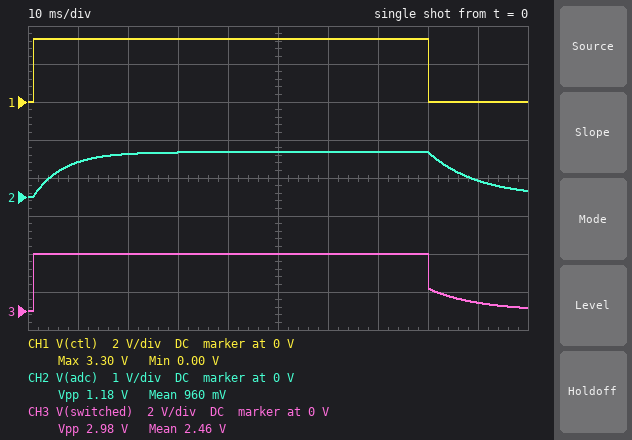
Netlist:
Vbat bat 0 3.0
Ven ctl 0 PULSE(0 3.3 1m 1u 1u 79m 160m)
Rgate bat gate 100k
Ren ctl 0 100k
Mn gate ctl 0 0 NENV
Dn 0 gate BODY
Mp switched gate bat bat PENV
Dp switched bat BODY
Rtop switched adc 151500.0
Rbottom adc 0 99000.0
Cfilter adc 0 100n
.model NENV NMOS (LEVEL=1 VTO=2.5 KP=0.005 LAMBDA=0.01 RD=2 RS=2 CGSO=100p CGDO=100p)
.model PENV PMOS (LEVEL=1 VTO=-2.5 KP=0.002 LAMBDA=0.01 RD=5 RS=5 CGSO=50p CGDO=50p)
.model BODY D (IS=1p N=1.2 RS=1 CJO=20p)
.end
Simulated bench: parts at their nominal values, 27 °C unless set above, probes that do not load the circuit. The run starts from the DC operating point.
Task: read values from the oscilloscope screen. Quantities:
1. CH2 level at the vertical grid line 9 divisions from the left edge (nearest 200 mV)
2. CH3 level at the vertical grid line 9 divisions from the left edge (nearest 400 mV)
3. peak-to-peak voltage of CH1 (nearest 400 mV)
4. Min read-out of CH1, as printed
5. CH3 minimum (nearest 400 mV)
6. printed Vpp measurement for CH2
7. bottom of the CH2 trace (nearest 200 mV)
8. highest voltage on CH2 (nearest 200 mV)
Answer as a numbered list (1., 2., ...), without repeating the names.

1. 400 mV
2. 400 mV
3. 3.2 V
4. 0.00 V
5. 0 V
6. 1.18 V
7. 0 V
8. 1.2 V
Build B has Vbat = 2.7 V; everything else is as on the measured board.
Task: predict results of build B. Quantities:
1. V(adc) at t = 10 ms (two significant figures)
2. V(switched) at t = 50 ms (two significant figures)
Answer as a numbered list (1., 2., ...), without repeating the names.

1. 820 mV
2. 2.7 V
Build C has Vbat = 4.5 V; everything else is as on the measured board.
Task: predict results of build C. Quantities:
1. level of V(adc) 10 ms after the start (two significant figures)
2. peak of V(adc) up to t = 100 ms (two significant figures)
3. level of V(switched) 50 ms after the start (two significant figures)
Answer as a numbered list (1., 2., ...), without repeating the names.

1. 1.4 V
2. 1.8 V
3. 4.5 V
